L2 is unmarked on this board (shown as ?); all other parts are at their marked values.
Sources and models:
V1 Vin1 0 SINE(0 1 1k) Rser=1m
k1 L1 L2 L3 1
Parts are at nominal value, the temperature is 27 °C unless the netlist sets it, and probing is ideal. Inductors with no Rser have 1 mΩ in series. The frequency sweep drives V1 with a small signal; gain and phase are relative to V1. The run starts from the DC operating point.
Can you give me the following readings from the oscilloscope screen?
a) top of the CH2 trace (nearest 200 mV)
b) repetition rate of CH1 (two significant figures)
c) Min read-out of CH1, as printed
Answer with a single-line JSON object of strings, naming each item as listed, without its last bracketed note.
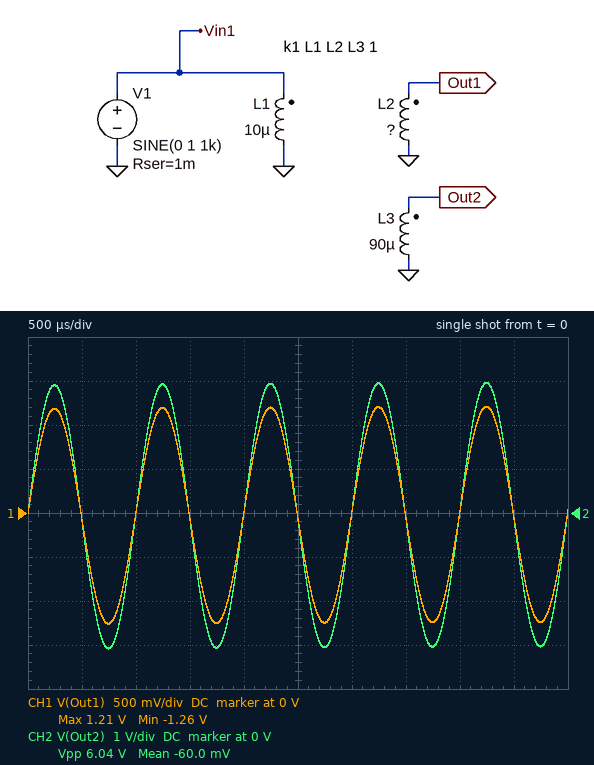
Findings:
{"top of the CH2 trace": "3.0 V", "repetition rate of CH1": "1.0 kHz", "Min read-out of CH1, as printed": "-1.26 V"}
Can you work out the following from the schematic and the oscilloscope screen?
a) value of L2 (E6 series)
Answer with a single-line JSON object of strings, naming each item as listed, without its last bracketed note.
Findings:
{"value of L2": "15 µH"}
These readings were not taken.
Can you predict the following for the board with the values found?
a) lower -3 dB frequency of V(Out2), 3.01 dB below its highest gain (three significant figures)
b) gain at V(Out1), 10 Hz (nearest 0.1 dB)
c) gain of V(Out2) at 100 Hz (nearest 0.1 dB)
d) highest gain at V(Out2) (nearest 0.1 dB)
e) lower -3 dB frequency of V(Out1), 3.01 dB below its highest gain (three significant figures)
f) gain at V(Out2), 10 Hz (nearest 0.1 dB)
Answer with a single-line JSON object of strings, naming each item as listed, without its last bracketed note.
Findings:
{"lower -3 dB frequency of V(Out2), 3.01 dB below its highest gain": "31.8 Hz", "gain at V(Out1), 10 Hz": "-8.7 dB", "gain of V(Out2) at 100 Hz": "9.1 dB", "highest gain at V(Out2)": "9.5 dB", "lower -3 dB frequency of V(Out1), 3.01 dB below its highest gain": "31.8 Hz", "gain at V(Out2), 10 Hz": "-0.9 dB"}
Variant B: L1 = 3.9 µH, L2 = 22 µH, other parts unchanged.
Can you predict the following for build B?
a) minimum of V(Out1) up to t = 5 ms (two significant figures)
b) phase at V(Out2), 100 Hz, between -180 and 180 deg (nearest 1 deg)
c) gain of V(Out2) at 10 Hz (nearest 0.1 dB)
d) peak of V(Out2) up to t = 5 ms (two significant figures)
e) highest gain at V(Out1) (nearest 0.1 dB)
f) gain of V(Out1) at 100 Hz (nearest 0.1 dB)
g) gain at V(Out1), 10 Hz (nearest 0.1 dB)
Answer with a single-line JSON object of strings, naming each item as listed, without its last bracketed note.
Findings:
{"minimum of V(Out1) up to t = 5 ms": "-2.5 V", "phase at V(Out2), 100 Hz, between -180 and 180 deg": "39 deg", "gain of V(Out2) at 10 Hz": "-4.7 dB", "peak of V(Out2) up to t = 5 ms": "4.7 V", "highest gain at V(Out1)": "7.5 dB", "gain of V(Out1) at 100 Hz": "5.3 dB", "gain at V(Out1), 10 Hz": "-10.8 dB"}
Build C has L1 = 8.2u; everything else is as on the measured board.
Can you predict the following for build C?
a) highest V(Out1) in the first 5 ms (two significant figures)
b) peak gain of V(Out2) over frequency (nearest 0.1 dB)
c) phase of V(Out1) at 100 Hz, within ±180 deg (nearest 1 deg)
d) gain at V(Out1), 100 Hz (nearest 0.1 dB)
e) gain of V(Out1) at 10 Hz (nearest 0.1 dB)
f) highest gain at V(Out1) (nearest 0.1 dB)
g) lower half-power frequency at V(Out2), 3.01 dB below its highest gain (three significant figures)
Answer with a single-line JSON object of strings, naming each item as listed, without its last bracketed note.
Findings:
{"highest V(Out1) in the first 5 ms": "1.3 V", "peak gain of V(Out2) over frequency": "10.4 dB", "phase of V(Out1) at 100 Hz, within ±180 deg": "21 deg", "gain at V(Out1), 100 Hz": "2.0 dB", "gain of V(Out1) at 10 Hz": "-9.4 dB", "highest gain at V(Out1)": "2.6 dB", "lower half-power frequency at V(Out2), 3.01 dB below its highest gain": "38.8 Hz"}
